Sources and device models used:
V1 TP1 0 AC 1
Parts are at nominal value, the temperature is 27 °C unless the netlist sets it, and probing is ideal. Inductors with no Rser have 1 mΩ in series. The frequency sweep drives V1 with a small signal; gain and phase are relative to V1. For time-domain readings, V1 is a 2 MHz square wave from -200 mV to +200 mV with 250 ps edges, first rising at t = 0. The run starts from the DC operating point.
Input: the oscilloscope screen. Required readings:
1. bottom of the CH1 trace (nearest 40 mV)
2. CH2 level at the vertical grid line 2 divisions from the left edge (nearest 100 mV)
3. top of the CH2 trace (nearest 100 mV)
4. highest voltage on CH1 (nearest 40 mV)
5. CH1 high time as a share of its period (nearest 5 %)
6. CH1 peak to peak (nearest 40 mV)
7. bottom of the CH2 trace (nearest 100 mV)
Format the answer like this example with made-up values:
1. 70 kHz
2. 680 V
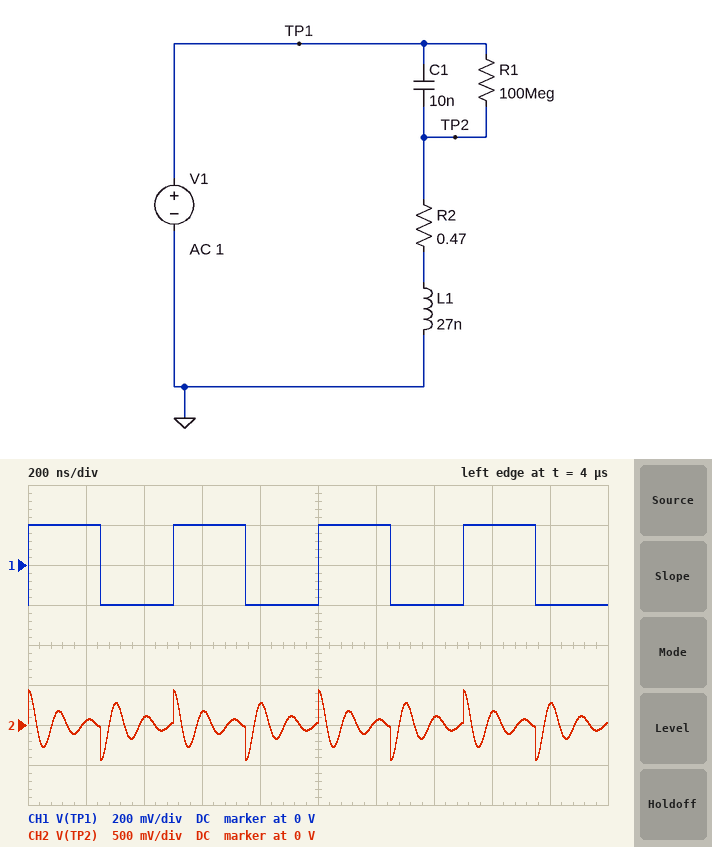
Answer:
1. -200 mV
2. 100 mV
3. 400 mV
4. 200 mV
5. 50 %
6. 400 mV
7. -400 mV
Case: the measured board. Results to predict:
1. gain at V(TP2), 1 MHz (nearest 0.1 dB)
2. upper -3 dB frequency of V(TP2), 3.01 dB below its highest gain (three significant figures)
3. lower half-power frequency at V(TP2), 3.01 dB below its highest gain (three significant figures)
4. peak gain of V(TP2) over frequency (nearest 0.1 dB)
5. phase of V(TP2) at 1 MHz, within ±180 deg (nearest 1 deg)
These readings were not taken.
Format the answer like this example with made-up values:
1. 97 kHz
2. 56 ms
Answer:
1. -30.0 dB
2. 11.7 MHz
3. 8.67 MHz
4. 11.3 dB
5. 108 deg
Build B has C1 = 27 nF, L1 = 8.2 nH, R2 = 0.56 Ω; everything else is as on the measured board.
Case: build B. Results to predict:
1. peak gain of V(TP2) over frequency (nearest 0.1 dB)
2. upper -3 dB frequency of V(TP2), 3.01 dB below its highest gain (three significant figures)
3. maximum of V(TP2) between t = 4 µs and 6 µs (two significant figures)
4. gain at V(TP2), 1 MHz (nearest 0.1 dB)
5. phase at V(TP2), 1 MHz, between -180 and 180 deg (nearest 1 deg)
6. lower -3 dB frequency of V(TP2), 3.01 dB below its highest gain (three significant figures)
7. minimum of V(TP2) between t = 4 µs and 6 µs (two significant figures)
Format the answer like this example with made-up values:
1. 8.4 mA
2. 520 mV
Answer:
1. 3.3 dB
2. 62.7 MHz
3. 400 mV
4. -20.4 dB
5. 90 deg
6. 7.73 MHz
7. -400 mV
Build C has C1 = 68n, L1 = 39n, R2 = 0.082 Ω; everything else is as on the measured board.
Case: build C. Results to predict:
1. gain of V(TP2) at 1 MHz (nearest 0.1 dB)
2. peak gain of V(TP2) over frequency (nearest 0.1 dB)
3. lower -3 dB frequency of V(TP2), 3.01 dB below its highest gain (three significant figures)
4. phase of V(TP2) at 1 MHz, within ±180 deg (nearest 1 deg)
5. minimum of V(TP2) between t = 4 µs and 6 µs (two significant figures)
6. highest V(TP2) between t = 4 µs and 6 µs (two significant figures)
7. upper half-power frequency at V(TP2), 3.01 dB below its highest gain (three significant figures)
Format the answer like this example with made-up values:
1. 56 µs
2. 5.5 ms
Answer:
1. -18.2 dB
2. 19.3 dB
3. 2.94 MHz
4. 159 deg
5. -260 mV
6. 260 mV
7. 3.29 MHz
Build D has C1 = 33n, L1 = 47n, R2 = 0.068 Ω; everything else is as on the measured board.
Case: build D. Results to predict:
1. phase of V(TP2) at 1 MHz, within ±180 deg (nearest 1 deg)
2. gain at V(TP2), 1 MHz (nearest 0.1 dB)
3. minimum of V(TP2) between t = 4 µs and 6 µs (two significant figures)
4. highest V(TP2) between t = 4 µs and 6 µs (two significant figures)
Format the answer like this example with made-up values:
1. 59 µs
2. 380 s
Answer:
1. 166 deg
2. -23.5 dB
3. -220 mV
4. 220 mV
